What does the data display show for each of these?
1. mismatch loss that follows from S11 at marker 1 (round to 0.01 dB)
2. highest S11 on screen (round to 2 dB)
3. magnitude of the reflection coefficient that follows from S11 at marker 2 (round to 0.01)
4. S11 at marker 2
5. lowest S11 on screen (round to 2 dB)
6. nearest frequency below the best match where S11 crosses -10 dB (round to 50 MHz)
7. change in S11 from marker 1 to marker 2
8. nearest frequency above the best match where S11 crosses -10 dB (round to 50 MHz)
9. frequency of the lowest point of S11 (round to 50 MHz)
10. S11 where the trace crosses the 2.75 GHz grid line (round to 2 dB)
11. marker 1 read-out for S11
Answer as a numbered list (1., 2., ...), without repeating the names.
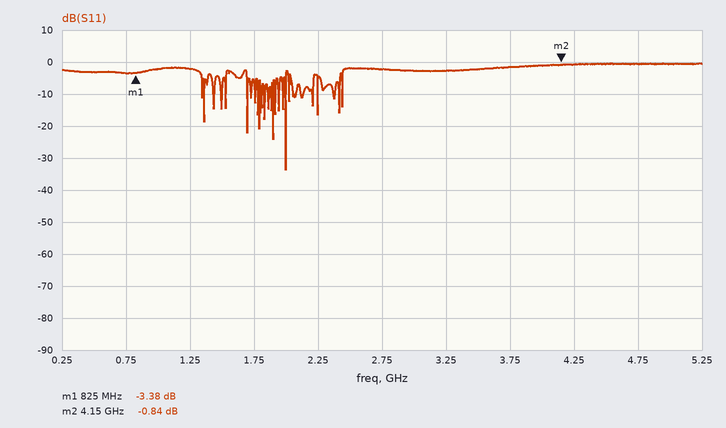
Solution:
1. 2.67 dB
2. 0 dB
3. 0.91
4. -0.84 dB
5. -34 dB
6. 2.00 GHz
7. 2.54 dB
8. 2.00 GHz
9. 2.00 GHz
10. -2 dB
11. -3.38 dB
